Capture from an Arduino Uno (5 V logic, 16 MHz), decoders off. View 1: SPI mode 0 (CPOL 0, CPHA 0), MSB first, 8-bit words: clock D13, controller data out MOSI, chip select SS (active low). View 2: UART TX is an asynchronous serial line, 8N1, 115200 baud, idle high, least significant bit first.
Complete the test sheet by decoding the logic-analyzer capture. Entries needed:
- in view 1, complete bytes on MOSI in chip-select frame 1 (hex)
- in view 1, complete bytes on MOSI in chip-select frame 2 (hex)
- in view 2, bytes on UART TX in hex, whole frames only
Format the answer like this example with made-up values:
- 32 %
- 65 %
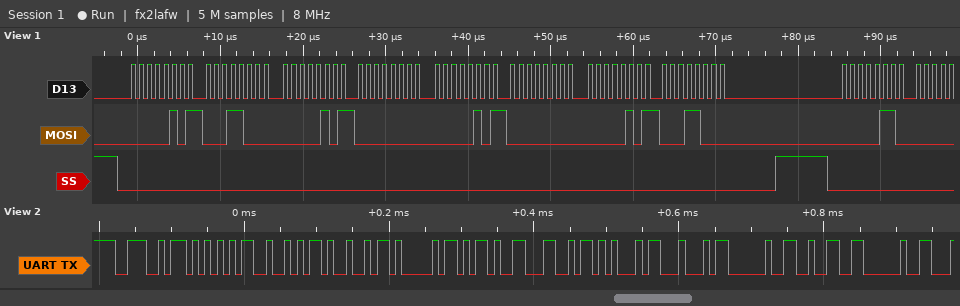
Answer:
- 05 18 05 00 05 00 05 18
- 06
- 4E 55 52 49 41 2D 4C 45 44 20 32 20
